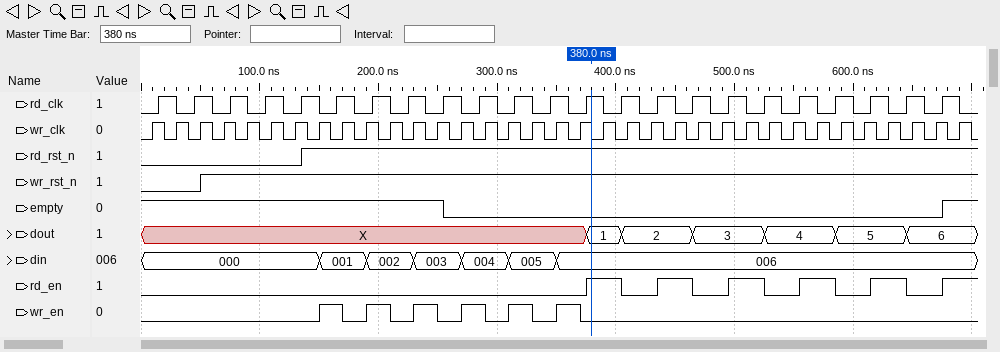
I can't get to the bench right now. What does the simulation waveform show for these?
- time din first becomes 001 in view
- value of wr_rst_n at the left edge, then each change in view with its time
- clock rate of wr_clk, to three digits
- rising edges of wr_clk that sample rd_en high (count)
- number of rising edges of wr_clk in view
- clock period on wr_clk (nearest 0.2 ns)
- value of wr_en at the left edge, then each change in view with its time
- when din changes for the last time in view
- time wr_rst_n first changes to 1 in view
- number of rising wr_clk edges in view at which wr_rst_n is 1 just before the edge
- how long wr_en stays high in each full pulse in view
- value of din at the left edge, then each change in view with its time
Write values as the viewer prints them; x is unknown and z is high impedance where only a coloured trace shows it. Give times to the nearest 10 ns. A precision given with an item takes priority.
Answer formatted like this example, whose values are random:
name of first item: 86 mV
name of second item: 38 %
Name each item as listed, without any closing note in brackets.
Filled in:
time din first becomes 001 in view: 150 ns
value of wr_rst_n at the left edge, then each change in view with its time: 0, 1 at 50 ns
clock rate of wr_clk, to three digits: 50.0 MHz
rising edges of wr_clk that sample rd_en high: 6
number of rising edges of wr_clk in view: 35
clock period on wr_clk: 20 ns
value of wr_en at the left edge, then each change in view with its time: 0, 1 at 150 ns, 0 at 170 ns, 1 at 190 ns, 0 at 210 ns, 1 at 230 ns, 0 at 250 ns, 1 at 270 ns, 0 at 290 ns, 1 at 310 ns, 0 at 330 ns, 1 at 350 ns, 0 at 370 ns
when din changes for the last time in view: 350 ns
time wr_rst_n first changes to 1 in view: 50 ns
number of rising wr_clk edges in view at which wr_rst_n is 1 just before the edge: 32
how long wr_en stays high in each full pulse in view: 20 ns, 20 ns, 20 ns, 20 ns, 20 ns, 20 ns
value of din at the left edge, then each change in view with its time: 000, 001 at 150 ns, 002 at 190 ns, 003 at 230 ns, 004 at 270 ns, 005 at 310 ns, 006 at 350 ns
